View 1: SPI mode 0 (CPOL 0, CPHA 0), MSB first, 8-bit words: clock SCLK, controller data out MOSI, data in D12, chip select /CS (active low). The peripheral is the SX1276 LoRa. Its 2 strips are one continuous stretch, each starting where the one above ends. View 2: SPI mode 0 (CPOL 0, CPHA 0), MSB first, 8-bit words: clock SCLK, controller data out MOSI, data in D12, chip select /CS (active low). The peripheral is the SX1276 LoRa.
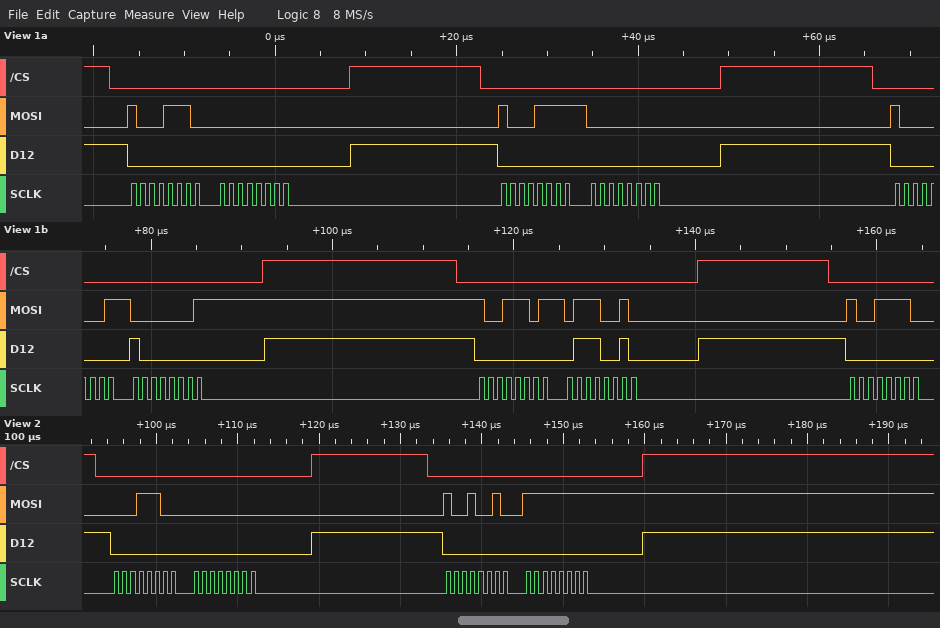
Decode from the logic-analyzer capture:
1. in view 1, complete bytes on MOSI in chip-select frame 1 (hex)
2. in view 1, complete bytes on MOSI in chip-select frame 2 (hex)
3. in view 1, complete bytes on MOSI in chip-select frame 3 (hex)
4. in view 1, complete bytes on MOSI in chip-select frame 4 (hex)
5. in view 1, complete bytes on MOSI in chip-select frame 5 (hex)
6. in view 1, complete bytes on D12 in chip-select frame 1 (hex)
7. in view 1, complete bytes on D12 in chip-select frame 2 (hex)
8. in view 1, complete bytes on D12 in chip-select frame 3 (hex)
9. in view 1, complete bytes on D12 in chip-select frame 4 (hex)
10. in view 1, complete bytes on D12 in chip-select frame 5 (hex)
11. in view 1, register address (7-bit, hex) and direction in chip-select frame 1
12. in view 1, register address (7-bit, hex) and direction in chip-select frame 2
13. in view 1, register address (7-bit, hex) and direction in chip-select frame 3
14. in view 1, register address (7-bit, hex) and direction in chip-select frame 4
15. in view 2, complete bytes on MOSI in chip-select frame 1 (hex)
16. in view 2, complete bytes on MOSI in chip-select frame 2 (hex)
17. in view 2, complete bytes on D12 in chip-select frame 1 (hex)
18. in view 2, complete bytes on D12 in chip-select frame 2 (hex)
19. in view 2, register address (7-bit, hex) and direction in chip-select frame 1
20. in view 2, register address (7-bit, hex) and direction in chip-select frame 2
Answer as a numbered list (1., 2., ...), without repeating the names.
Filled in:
1. 0x8E 0x00
2. 0x8F 0x00
3. 0x81 0x01
4. 0x9D 0x72
5. 0x9E
6. 0x00 0x00
7. 0x00 0x00
8. 0x00 0x80
9. 0x00 0x72
10. 0x00
11. 0x0E write
12. 0x0F write
13. 0x01 write
14. 0x1D write
15. 1C 00
16. 92 FF
17. 00 00
18. 00 00
19. 0x1C read
20. 0x12 write
